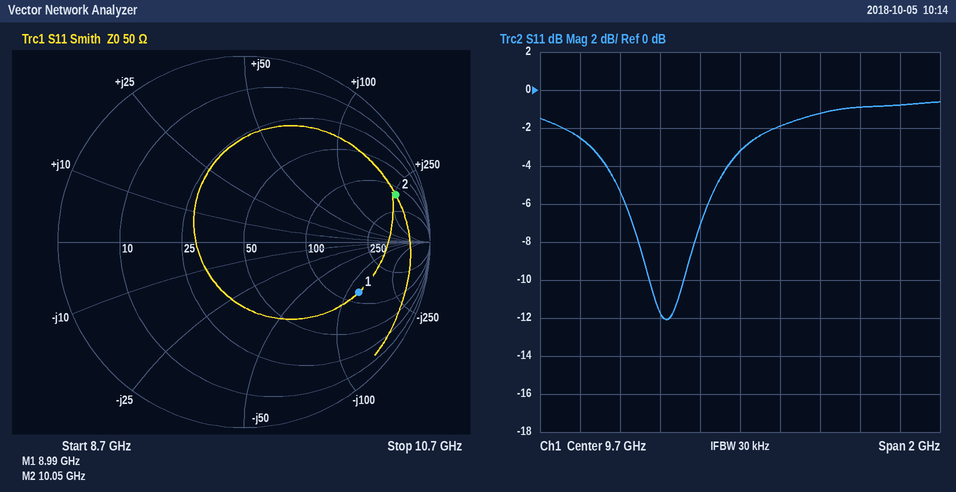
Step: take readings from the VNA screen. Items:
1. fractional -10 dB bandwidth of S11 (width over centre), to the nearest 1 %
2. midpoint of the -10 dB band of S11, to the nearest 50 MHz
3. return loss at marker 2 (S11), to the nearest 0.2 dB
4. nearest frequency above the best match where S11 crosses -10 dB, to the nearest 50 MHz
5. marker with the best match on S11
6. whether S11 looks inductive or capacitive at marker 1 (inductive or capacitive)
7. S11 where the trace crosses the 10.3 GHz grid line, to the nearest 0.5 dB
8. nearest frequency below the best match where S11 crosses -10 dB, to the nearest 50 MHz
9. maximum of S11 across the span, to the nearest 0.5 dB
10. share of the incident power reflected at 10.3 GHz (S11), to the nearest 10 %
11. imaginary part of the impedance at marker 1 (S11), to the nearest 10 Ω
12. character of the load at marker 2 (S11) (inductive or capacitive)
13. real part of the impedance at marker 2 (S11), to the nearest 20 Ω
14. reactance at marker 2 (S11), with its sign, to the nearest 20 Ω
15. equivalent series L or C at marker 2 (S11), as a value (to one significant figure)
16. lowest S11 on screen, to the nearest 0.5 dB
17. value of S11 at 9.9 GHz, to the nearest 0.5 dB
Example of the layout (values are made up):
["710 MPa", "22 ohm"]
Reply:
["2 %", "9.35 GHz", "1.4 dB", "9.40 GHz", "marker 1", "capacitive", "-1.0 dB", "9.25 GHz", "-0.5 dB", "80 %", "-120 Ω", "inductive", "140 Ω", "+260 Ω", "4 nH", "-12.0 dB", "-2.0 dB"]
